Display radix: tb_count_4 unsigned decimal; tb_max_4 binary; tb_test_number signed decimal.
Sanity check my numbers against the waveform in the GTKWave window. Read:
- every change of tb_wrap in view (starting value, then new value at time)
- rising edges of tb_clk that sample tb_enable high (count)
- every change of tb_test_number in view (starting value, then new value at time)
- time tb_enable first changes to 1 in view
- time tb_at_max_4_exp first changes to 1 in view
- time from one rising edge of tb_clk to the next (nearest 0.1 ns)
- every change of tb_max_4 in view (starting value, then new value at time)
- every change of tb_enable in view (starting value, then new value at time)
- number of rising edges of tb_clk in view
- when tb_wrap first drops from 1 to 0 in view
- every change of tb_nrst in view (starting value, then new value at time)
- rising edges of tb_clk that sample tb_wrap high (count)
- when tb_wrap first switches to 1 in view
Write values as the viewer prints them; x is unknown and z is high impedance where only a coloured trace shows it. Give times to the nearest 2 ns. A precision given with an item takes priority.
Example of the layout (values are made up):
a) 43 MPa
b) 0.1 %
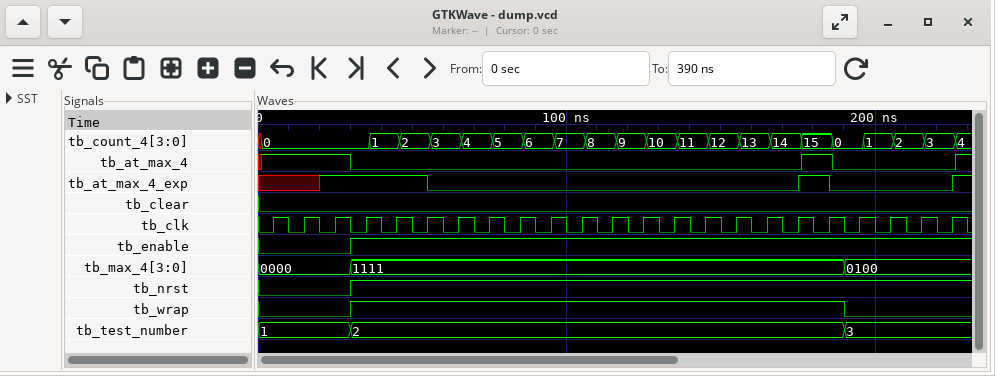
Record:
a) 0, 1 at 30 ns, 0 at 190 ns
b) 20
c) 1, 2 at 30 ns, 3 at 190 ns
d) 30 ns
e) 20 ns
f) 10 ns
g) 0000, 1111 at 30 ns, 0100 at 190 ns
h) 0, 1 at 30 ns
i) 23
j) 190 ns
k) 0, 1 at 30 ns
l) 16
m) 30 ns
